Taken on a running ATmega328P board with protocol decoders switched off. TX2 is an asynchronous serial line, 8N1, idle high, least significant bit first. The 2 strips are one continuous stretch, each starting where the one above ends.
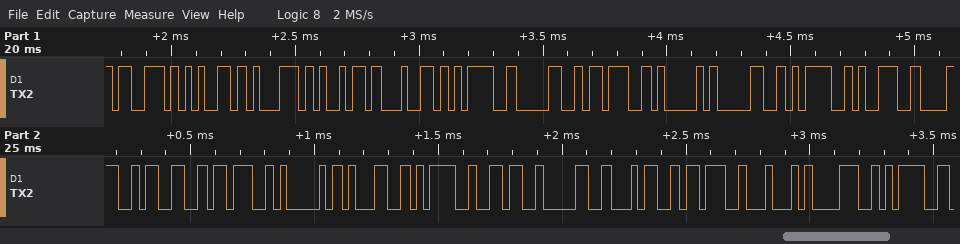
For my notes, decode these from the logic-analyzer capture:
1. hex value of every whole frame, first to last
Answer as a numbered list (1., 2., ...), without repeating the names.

1. 0x73 0x65 0x71 0x69 0x64 0x3D 0x30 0x3B 0x41 0x30 0x3D 0x39 0x38 0x33 0x3B 0x41 0x31 0x3D 0x36 0x30 0x34 0x3B 0x44 0x38 0x3D
